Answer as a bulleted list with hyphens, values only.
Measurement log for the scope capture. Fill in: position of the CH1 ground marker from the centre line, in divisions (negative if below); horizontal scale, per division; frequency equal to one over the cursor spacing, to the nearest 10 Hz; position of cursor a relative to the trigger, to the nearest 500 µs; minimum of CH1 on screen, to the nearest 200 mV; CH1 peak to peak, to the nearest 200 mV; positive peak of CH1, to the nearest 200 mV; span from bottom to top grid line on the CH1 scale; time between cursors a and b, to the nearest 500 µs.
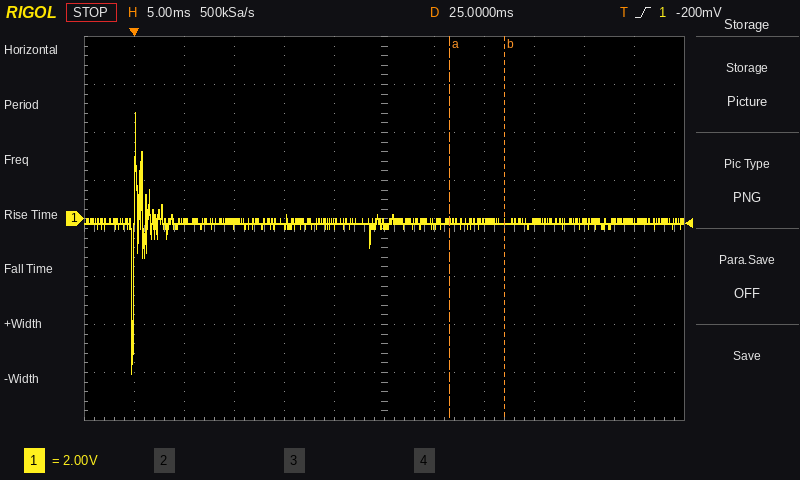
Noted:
- +0.2 div
- 5 ms
- 180 Hz
- +31.5 ms
- -6.4 V
- 10.8 V
- 4.4 V
- 16 V
- 5.5 ms
